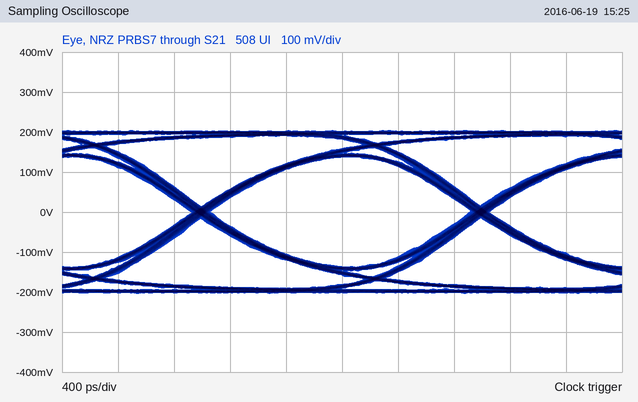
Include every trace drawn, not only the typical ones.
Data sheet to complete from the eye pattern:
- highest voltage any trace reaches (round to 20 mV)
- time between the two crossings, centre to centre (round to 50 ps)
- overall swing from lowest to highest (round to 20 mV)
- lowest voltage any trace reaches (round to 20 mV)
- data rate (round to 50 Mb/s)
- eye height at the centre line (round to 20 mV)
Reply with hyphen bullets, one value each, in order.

- 200 mV
- 2.00 ns
- 400 mV
- -200 mV
- 500 Mb/s
- 280 mV
